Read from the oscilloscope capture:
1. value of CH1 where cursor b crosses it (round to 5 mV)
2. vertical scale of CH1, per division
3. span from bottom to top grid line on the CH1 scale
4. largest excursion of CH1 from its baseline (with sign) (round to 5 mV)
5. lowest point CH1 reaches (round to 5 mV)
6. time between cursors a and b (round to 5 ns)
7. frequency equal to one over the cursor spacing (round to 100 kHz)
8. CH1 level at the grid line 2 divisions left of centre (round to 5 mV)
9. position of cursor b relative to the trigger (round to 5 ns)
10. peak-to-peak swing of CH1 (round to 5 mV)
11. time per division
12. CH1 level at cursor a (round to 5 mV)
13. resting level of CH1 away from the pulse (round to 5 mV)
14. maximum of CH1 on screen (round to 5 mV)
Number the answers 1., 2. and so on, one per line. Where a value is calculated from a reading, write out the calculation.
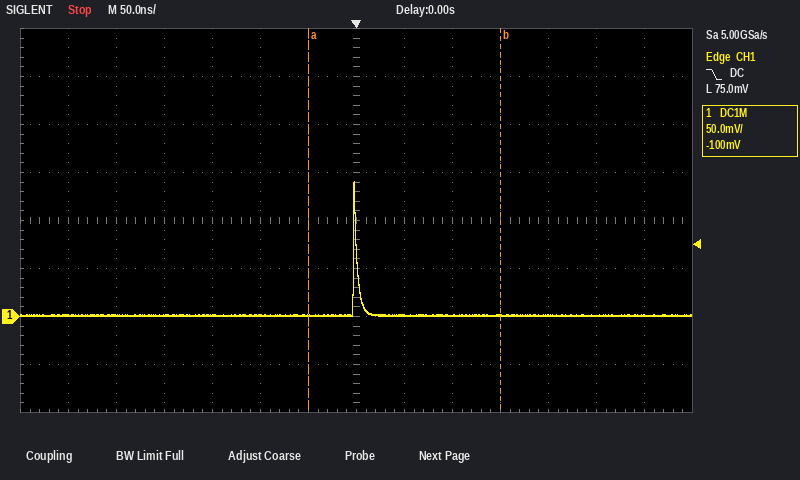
1. 0 mV
2. 50 mV
3. 400 mV
4. 140 mV − (0 mV) = +140 mV
5. 0 mV
6. 200 ns
7. 1 / 200 ns ≈ 5.0 MHz
8. 0 mV
9. +150 ns
10. 140 mV − (0 mV) = 140 mV
11. 50 ns
12. 0 mV
13. 0 mV
14. 140 mV
